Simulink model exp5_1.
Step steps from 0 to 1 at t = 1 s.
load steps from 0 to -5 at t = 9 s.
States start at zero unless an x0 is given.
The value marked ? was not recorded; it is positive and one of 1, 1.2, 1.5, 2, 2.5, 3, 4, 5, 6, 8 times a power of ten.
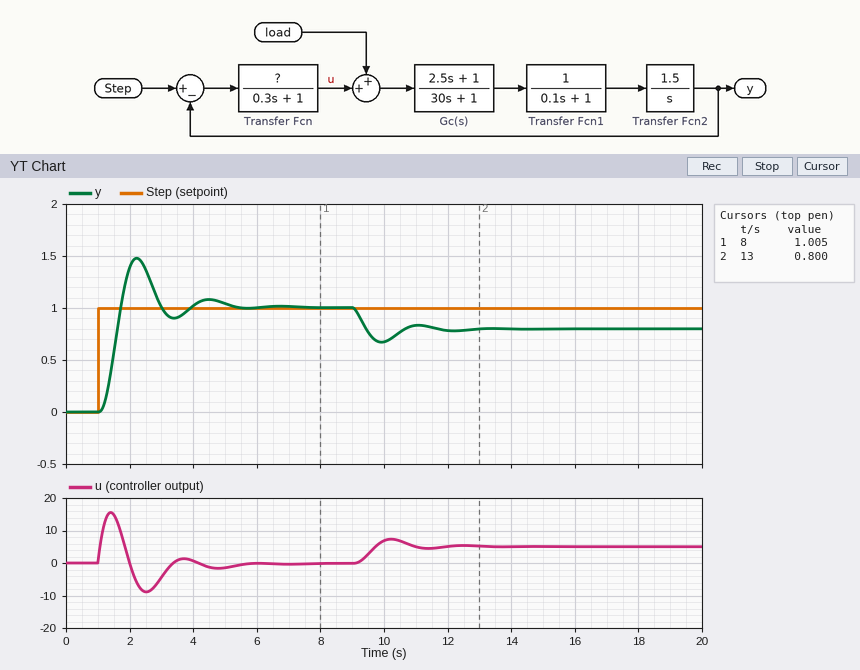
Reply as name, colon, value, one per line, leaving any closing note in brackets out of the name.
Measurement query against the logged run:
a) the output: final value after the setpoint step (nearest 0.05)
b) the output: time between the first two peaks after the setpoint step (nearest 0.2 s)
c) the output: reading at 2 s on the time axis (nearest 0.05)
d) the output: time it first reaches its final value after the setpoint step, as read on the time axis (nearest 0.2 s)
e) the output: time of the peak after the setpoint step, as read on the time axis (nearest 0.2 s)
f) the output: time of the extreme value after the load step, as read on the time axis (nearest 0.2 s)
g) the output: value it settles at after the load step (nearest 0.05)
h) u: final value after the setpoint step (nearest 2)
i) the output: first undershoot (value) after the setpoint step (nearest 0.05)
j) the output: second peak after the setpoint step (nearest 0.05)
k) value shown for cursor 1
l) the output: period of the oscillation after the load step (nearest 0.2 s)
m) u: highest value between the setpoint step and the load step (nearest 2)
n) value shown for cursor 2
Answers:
the output: final value after the setpoint step: 1.00
the output: time between the first two peaks after the setpoint step: 2.2 s
the output: reading at 2 s on the time axis: 1.40
the output: time it first reaches its final value after the setpoint step, as read on the time axis: 1.8 s
the output: time of the peak after the setpoint step, as read on the time axis: 2.2 s
the output: time of the extreme value after the load step, as read on the time axis: 10.0 s
the output: value it settles at after the load step: 0.80
u: final value after the setpoint step: 0
the output: first undershoot (value) after the setpoint step: 0.90
the output: second peak after the setpoint step: 1.10
value shown for cursor 1: 1.005
the output: period of the oscillation after the load step: 2.2 s
u: highest value between the setpoint step and the load step: 16
value shown for cursor 2: 0.800
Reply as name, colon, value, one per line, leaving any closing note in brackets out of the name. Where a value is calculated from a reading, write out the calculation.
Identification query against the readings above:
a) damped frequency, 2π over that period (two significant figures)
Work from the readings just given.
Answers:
damped frequency, 2π over that period: 2π / 2.2 = 2.9 rad/s
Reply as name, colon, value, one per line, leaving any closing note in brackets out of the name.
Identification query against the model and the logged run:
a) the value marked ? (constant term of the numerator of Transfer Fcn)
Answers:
the value marked ?: 25
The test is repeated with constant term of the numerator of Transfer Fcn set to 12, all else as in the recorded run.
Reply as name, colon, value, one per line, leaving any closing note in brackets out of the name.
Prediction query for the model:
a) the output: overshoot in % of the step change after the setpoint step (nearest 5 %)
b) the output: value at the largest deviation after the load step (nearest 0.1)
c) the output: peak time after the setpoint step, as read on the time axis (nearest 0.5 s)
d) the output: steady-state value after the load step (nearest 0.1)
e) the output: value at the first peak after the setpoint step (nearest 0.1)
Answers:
the output: overshoot in % of the step change after the setpoint step: 30 %
the output: value at the largest deviation after the load step: 0.4
the output: peak time after the setpoint step, as read on the time axis: 3.0 s
the output: steady-state value after the load step: 0.6
the output: value at the first peak after the setpoint step: 1.3
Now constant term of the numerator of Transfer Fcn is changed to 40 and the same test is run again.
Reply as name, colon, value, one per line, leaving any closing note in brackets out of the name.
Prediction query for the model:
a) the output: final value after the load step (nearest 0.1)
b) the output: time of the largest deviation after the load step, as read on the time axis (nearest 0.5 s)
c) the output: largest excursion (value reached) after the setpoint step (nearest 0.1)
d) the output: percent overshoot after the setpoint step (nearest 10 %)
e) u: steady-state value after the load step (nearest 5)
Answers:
the output: final value after the load step: 0.9
the output: time of the largest deviation after the load step, as read on the time axis: 9.5 s
the output: largest excursion (value reached) after the setpoint step: 1.6
the output: percent overshoot after the setpoint step: 60 %
u: steady-state value after the load step: 5
